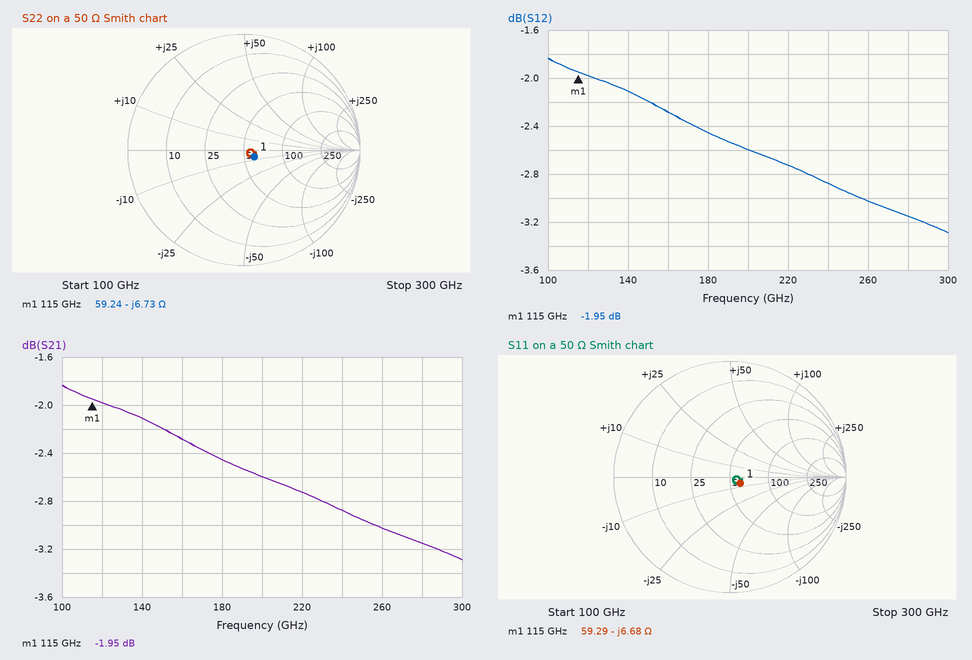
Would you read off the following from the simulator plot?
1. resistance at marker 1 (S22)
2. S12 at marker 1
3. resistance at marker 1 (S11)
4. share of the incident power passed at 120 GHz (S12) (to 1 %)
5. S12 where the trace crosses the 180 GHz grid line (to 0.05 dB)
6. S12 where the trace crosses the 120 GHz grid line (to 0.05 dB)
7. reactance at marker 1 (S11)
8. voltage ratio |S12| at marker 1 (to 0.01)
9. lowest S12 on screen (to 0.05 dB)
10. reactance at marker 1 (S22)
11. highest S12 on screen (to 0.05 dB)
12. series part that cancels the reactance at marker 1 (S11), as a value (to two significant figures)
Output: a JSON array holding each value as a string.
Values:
["59.24 Ω", "-1.95 dB", "59.29 Ω", "63 %", "-2.45 dB", "-2.00 dB", "-6.68 Ω", "0.80", "-3.30 dB", "-6.73 Ω", "-1.85 dB", "9.2 pH"]
